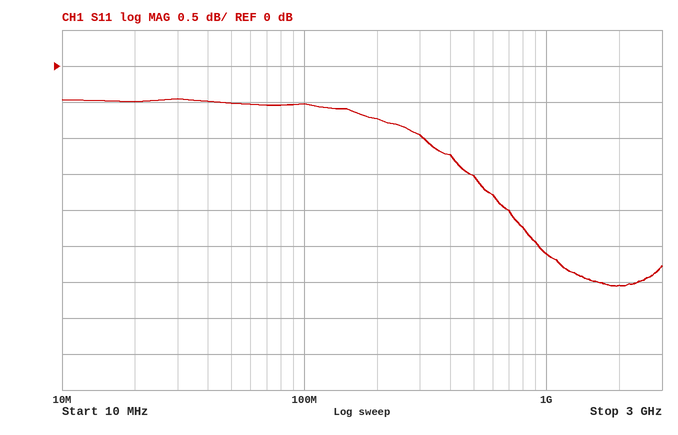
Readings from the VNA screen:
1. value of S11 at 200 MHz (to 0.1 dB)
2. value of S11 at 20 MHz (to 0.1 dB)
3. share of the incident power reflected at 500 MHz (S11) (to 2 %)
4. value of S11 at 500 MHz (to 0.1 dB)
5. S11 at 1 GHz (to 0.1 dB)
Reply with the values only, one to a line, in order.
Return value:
-0.7 dB
-0.5 dB
70 %
-1.5 dB
-2.6 dB
